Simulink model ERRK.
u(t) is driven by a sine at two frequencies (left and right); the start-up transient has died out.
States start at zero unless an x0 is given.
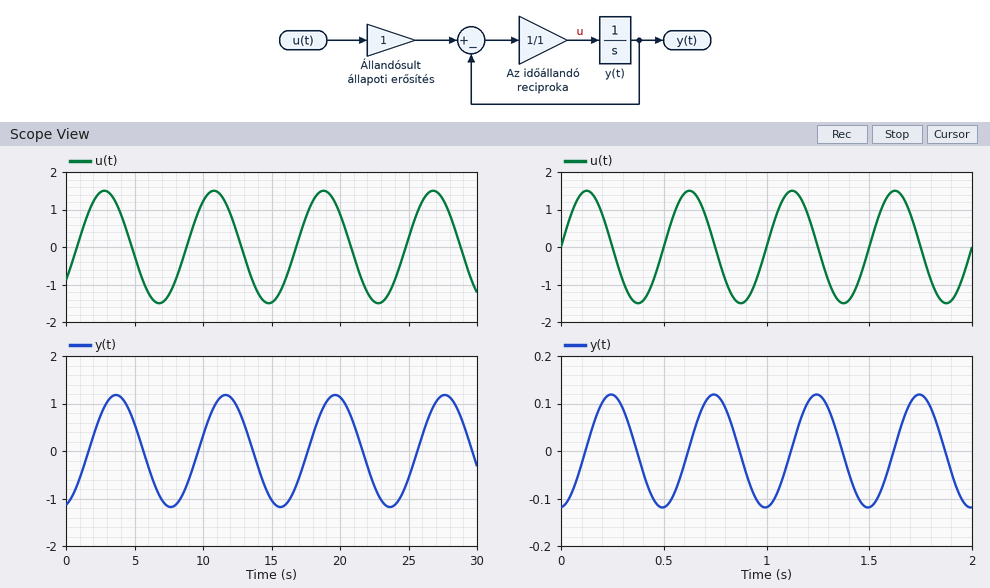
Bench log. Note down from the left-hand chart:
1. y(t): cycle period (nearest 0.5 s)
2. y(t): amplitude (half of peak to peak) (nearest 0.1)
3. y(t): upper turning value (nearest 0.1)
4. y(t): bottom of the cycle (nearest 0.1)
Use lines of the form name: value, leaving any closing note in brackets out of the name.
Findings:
y(t): cycle period: 8.0 s
y(t): amplitude (half of peak to peak): 1.2
y(t): upper turning value: 1.2
y(t): bottom of the cycle: -1.2
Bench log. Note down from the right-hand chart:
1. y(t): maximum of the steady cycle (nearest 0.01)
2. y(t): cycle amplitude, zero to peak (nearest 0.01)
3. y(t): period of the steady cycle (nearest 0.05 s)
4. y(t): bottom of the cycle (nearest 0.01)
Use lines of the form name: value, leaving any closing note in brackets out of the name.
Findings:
y(t): maximum of the steady cycle: 0.12
y(t): cycle amplitude, zero to peak: 0.12
y(t): period of the steady cycle: 0.50 s
y(t): bottom of the cycle: -0.12
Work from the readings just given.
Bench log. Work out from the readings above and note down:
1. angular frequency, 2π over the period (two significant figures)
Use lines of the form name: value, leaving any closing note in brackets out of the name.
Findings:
angular frequency, 2π over the period: 13 rad/s
